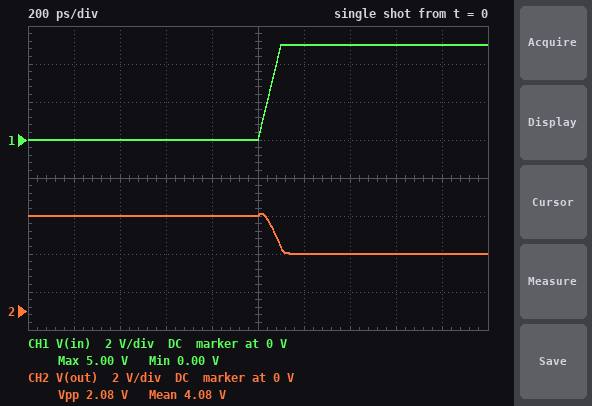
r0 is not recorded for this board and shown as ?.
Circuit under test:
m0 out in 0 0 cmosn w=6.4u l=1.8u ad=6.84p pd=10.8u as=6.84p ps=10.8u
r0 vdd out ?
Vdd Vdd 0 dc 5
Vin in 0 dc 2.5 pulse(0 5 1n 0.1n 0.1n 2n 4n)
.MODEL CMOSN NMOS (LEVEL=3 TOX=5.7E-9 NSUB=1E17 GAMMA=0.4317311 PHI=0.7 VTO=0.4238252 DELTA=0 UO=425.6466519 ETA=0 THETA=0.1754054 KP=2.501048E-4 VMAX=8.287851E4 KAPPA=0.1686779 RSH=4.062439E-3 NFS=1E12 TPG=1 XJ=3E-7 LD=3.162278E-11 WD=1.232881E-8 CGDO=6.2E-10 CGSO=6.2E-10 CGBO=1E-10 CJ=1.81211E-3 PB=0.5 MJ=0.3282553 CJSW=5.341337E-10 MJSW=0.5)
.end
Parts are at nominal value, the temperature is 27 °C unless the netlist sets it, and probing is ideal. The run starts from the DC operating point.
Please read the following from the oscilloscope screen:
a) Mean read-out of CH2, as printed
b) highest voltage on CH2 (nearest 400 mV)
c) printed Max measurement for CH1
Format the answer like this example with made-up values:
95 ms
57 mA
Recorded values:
4.08 V
5.2 V
5.00 V
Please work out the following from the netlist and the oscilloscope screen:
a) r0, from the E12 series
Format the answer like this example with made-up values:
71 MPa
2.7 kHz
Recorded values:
680 Ω
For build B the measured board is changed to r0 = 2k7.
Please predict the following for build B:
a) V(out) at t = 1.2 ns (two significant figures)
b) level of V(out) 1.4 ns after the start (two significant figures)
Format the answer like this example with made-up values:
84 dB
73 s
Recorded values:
890 mV
860 mV
